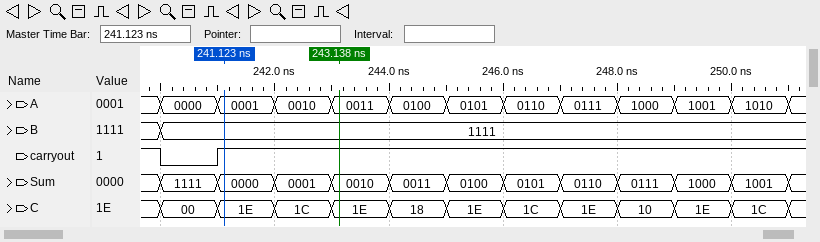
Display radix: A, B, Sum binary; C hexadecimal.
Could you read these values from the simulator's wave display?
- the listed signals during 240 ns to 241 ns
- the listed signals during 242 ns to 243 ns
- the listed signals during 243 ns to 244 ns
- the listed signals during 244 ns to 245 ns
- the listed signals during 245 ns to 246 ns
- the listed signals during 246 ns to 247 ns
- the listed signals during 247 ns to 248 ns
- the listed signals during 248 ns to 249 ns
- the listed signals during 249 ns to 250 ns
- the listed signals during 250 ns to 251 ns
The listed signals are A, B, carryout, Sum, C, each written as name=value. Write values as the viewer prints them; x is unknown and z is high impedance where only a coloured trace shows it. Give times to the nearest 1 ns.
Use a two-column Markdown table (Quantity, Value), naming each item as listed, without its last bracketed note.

| Quantity | Value |
|---|---|
| the listed signals during 240 ns to 241 ns | A=0000, B=1111, carryout=0, Sum=1111, C=00 |
| the listed signals during 242 ns to 243 ns | A=0010, B=1111, carryout=1, Sum=0001, C=1C |
| the listed signals during 243 ns to 244 ns | A=0011, B=1111, carryout=1, Sum=0010, C=1E |
| the listed signals during 244 ns to 245 ns | A=0100, B=1111, carryout=1, Sum=0011, C=18 |
| the listed signals during 245 ns to 246 ns | A=0101, B=1111, carryout=1, Sum=0100, C=1E |
| the listed signals during 246 ns to 247 ns | A=0110, B=1111, carryout=1, Sum=0101, C=1C |
| the listed signals during 247 ns to 248 ns | A=0111, B=1111, carryout=1, Sum=0110, C=1E |
| the listed signals during 248 ns to 249 ns | A=1000, B=1111, carryout=1, Sum=0111, C=10 |
| the listed signals during 249 ns to 250 ns | A=1001, B=1111, carryout=1, Sum=1000, C=1E |
| the listed signals during 250 ns to 251 ns | A=1010, B=1111, carryout=1, Sum=1001, C=1C |
